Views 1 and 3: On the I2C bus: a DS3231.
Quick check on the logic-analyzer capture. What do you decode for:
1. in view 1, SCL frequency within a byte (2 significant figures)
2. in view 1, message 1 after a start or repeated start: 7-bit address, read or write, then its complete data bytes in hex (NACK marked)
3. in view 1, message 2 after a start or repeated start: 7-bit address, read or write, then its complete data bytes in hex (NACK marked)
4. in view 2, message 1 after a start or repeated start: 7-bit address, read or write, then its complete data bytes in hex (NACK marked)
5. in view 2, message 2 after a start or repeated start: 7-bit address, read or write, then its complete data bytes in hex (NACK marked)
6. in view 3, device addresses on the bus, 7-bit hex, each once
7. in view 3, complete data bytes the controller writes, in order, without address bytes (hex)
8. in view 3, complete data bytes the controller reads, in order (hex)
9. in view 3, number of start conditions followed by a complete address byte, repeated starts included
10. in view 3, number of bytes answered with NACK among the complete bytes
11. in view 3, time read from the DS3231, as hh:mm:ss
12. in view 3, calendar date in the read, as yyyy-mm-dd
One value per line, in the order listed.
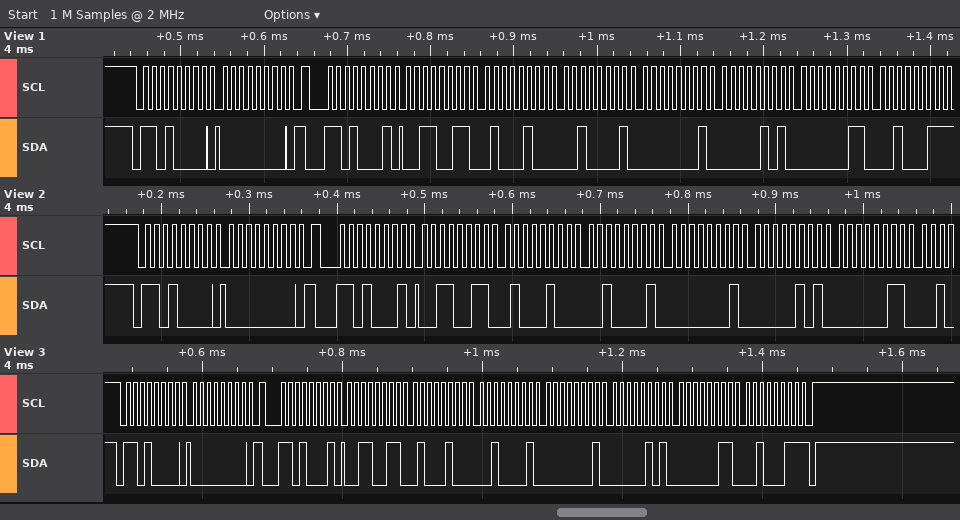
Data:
100 kHz
0x68 write: 00
0x68 read: 33 44 21 01 05 03 23 NACK
0x68 write: 00
0x68 read: 33 44 21 01 05 03
0x68
00
33 44 21 01 05 03 23
2
1
21:44:33
2023-03-05
